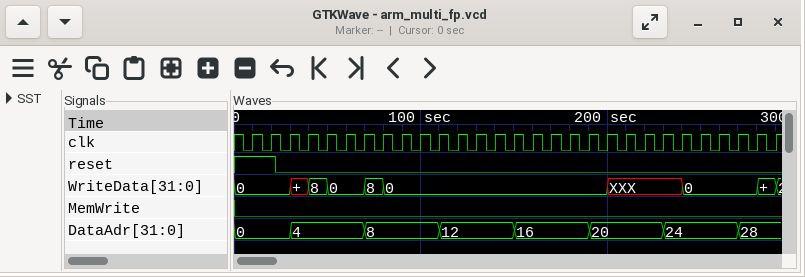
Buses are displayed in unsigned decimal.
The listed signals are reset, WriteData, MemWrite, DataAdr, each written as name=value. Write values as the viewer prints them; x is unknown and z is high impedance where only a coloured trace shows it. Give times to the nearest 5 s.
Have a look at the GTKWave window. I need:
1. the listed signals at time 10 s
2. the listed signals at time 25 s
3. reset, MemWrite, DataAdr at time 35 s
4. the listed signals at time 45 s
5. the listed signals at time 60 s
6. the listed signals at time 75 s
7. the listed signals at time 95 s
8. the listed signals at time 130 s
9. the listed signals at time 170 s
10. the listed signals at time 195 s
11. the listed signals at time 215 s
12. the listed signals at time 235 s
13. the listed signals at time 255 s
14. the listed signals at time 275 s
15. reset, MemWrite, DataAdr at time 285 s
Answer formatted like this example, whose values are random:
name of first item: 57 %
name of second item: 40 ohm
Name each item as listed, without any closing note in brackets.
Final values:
the listed signals at time 10 s: reset=1, WriteData=0, MemWrite=0, DataAdr=0
the listed signals at time 25 s: reset=0, WriteData=0, MemWrite=0, DataAdr=0
reset, MemWrite, DataAdr at time 35 s: reset=0, MemWrite=0, DataAdr=4
the listed signals at time 45 s: reset=0, WriteData=8, MemWrite=0, DataAdr=4
the listed signals at time 60 s: reset=0, WriteData=0, MemWrite=0, DataAdr=4
the listed signals at time 75 s: reset=0, WriteData=8, MemWrite=0, DataAdr=8
the listed signals at time 95 s: reset=0, WriteData=0, MemWrite=0, DataAdr=8
the listed signals at time 130 s: reset=0, WriteData=0, MemWrite=0, DataAdr=12
the listed signals at time 170 s: reset=0, WriteData=0, MemWrite=0, DataAdr=16
the listed signals at time 195 s: reset=0, WriteData=0, MemWrite=0, DataAdr=20
the listed signals at time 215 s: reset=0, WriteData=XXX, MemWrite=0, DataAdr=20
the listed signals at time 235 s: reset=0, WriteData=XXX, MemWrite=0, DataAdr=24
the listed signals at time 255 s: reset=0, WriteData=0, MemWrite=0, DataAdr=24
the listed signals at time 275 s: reset=0, WriteData=0, MemWrite=0, DataAdr=28
reset, MemWrite, DataAdr at time 285 s: reset=0, MemWrite=0, DataAdr=28
